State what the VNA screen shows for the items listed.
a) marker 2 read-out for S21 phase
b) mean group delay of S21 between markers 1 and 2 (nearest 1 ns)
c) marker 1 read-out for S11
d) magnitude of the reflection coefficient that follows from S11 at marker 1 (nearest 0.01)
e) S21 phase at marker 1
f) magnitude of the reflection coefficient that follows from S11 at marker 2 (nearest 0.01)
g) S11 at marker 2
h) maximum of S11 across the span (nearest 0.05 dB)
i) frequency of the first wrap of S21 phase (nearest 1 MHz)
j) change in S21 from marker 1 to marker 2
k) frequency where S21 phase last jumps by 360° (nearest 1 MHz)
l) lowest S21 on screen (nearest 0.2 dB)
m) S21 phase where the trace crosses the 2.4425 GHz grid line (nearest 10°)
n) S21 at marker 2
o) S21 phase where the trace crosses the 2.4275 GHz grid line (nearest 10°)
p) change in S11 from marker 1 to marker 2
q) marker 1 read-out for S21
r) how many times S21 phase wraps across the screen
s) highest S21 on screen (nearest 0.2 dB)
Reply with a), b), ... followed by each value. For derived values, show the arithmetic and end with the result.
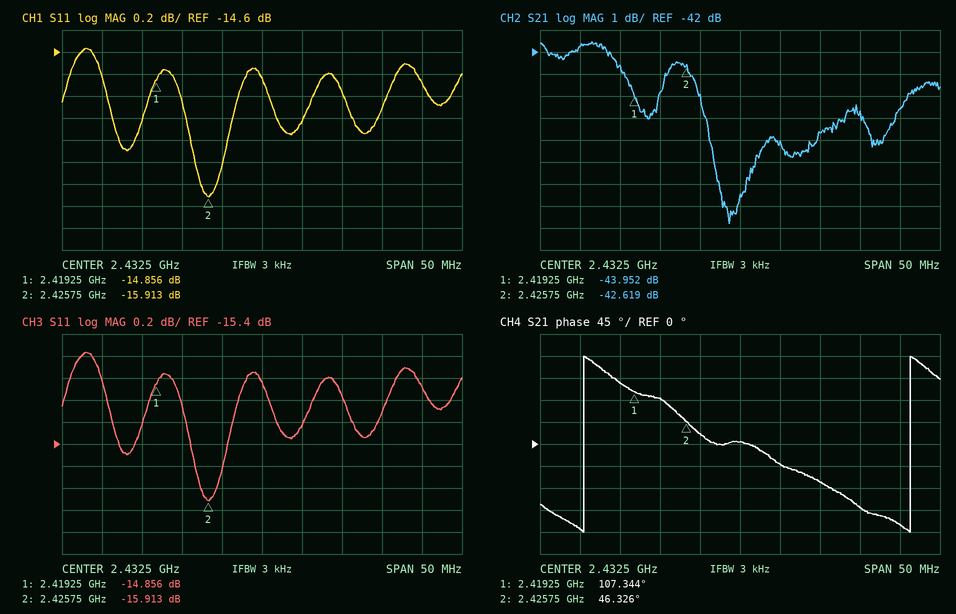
a) 46.326°
b) −(46.326° − (107.344°))/(360° × 6.5 MHz) ≈ 26 ns
c) -14.856 dB
d) 10^(-14.856/20) ≈ 0.18
e) 107.344°
f) 10^(-15.913/20) ≈ 0.16
g) -15.913 dB
h) -14.55 dB
i) 2.413 GHz
j) -42.619 − (-43.952) = 1.333 dB
k) 2.454 GHz
l) -49.8 dB
m) -80°
n) -42.619 dB
o) 20°
p) -15.913 − (-14.856) = -1.057 dB
q) -43.952 dB
r) 2
s) -41.6 dB
